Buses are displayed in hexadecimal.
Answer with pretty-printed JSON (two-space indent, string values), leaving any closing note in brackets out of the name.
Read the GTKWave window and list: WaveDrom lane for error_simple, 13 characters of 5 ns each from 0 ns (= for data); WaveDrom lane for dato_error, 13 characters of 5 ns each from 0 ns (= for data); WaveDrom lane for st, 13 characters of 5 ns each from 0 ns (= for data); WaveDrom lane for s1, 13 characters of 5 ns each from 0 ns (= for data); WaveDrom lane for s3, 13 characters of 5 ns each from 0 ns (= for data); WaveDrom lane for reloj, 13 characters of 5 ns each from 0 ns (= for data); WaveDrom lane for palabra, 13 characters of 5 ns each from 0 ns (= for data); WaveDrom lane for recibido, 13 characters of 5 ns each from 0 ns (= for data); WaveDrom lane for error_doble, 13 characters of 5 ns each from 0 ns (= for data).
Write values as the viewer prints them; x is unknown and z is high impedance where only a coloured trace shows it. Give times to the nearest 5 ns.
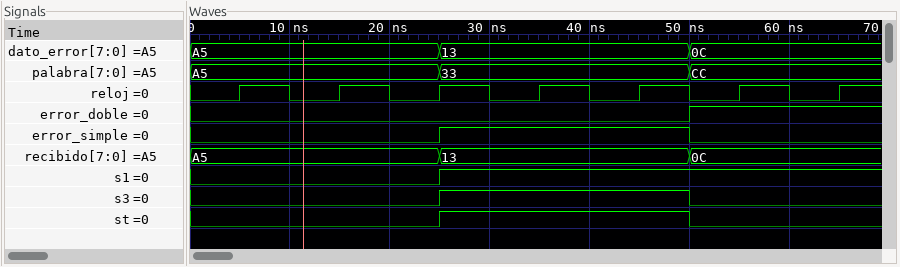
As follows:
{
  "WaveDrom lane for error_simple, 13 characters of 5 ns each from 0 ns": "{name: 'error_simple', wave: '0....1....0..'}",
  "WaveDrom lane for dato_error, 13 characters of 5 ns each from 0 ns": "{name: 'dato_error', wave: '=....=....=..', data: 'A5 13 0C'}",
  "WaveDrom lane for st, 13 characters of 5 ns each from 0 ns": "{name: 'st', wave: '0....1....0..'}",
  "WaveDrom lane for s1, 13 characters of 5 ns each from 0 ns": "{name: 's1', wave: '0....1.......'}",
  "WaveDrom lane for s3, 13 characters of 5 ns each from 0 ns": "{name: 's3', wave: '0....1....0..'}",
  "WaveDrom lane for reloj, 13 characters of 5 ns each from 0 ns": "{name: 'reloj', wave: '0101010101010'}",
  "WaveDrom lane for palabra, 13 characters of 5 ns each from 0 ns": "{name: 'palabra', wave: '=....=....=..', data: 'A5 33 CC'}",
  "WaveDrom lane for recibido, 13 characters of 5 ns each from 0 ns": "{name: 'recibido', wave: '=....=....=..', data: 'A5 13 0C'}",
  "WaveDrom lane for error_doble, 13 characters of 5 ns each from 0 ns": "{name: 'error_doble', wave: '0.........1..'}"
}
